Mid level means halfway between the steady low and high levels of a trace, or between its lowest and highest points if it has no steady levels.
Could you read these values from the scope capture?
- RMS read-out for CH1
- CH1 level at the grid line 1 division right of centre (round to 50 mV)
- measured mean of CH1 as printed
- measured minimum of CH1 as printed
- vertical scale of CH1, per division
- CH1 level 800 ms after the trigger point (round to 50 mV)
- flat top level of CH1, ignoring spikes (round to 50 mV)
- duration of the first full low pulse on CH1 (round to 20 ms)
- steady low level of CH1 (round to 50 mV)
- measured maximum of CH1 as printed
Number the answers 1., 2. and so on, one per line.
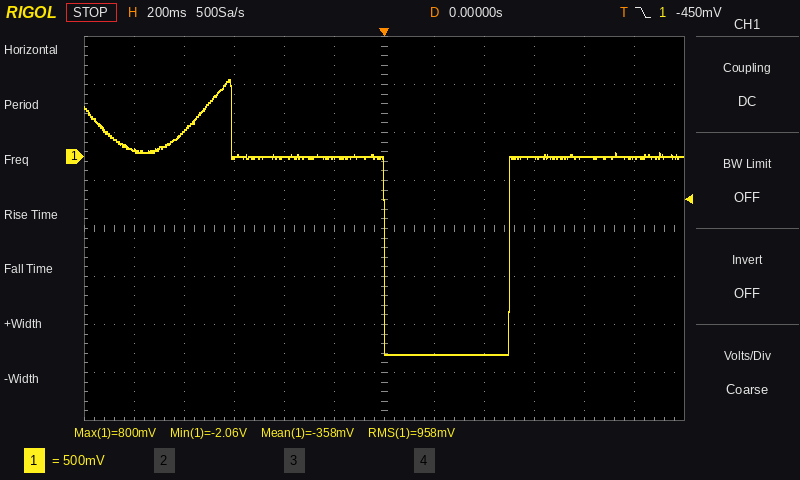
1. 958 mV
2. -2.05 V
3. -358 mV
4. -2.06 V
5. 500 mV
6. 0 mV
7. 0 mV
8. 500 ms
9. -2.05 V
10. 800 mV
